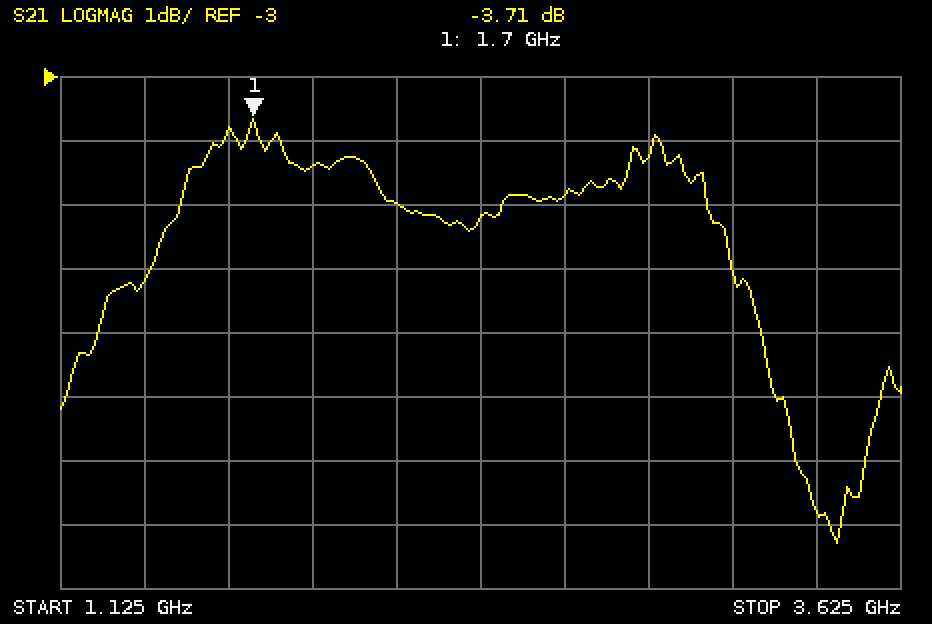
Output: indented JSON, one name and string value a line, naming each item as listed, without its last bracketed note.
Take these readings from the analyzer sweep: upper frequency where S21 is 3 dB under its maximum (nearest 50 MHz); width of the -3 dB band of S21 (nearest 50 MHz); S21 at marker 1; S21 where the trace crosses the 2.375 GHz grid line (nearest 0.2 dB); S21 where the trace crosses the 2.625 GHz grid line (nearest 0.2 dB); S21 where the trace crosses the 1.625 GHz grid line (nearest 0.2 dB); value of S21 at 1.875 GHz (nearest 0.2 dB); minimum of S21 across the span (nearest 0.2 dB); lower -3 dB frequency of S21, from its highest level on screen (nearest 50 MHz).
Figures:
{
  "upper frequency where S21 is 3 dB under its maximum": "3.20 GHz",
  "width of the -3 dB band of S21": "1.95 GHz",
  "S21 at marker 1": "-3.71 dB",
  "S21 where the trace crosses the 2.375 GHz grid line": "-5.2 dB",
  "S21 where the trace crosses the 2.625 GHz grid line": "-4.8 dB",
  "S21 where the trace crosses the 1.625 GHz grid line": "-3.8 dB",
  "value of S21 at 1.875 GHz": "-4.4 dB",
  "minimum of S21 across the span": "-10.2 dB",
  "lower -3 dB frequency of S21, from its highest level on screen": "1.25 GHz"
}
